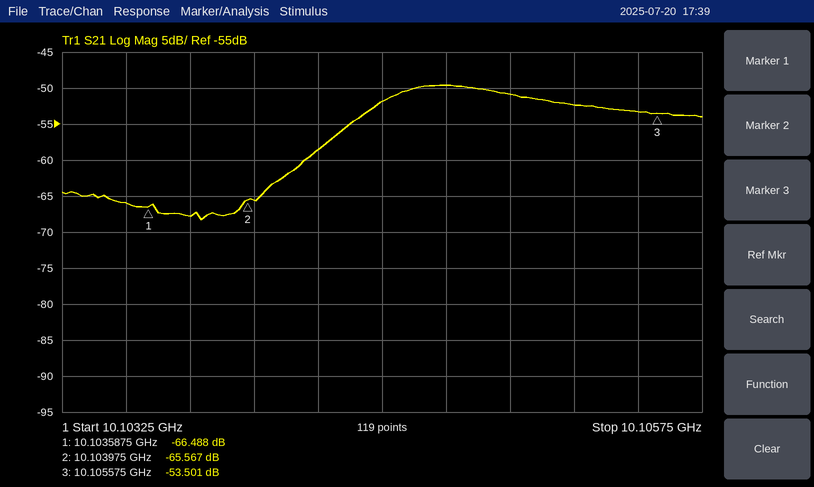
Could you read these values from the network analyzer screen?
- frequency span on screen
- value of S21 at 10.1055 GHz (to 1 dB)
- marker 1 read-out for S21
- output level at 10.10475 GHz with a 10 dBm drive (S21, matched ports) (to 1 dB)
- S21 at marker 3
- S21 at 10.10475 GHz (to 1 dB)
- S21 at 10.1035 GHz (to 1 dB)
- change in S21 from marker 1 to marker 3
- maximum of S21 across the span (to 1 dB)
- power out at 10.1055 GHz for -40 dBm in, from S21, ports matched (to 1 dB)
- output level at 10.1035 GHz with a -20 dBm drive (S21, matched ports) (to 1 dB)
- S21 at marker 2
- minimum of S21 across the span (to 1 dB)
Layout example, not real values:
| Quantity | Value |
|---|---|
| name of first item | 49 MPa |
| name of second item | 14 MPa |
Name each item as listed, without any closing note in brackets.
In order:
| Quantity | Value |
|---|---|
| frequency span on screen | 2.5 MHz |
| value of S21 at 10.1055 GHz | -53 dB |
| marker 1 read-out for S21 | -66.488 dB |
| output level at 10.10475 GHz with a 10 dBm drive (S21, matched ports) | -40 dBm |
| S21 at marker 3 | -53.501 dB |
| S21 at 10.10475 GHz | -50 dB |
| S21 at 10.1035 GHz | -66 dB |
| change in S21 from marker 1 to marker 3 | 12.987 dB |
| maximum of S21 across the span | -50 dB |
| power out at 10.1055 GHz for -40 dBm in, from S21, ports matched | -93 dBm |
| output level at 10.1035 GHz with a -20 dBm drive (S21, matched ports) | -86 dBm |
| S21 at marker 2 | -65.567 dB |
| minimum of S21 across the span | -68 dB |
